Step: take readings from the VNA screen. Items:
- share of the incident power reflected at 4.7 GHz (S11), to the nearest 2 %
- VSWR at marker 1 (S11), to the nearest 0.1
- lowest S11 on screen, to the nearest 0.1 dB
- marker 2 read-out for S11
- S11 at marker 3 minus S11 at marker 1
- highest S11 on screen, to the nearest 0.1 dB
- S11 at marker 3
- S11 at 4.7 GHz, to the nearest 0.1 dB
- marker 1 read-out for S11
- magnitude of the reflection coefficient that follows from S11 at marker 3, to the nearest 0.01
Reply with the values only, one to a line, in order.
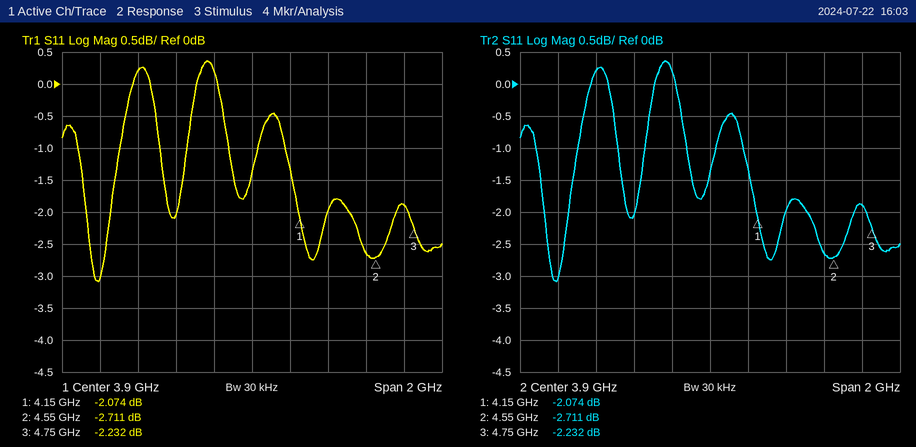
64 %
8.4
-3.1 dB
-2.711 dB
-0.158 dB
0.4 dB
-2.232 dB
-1.9 dB
-2.074 dB
0.77
